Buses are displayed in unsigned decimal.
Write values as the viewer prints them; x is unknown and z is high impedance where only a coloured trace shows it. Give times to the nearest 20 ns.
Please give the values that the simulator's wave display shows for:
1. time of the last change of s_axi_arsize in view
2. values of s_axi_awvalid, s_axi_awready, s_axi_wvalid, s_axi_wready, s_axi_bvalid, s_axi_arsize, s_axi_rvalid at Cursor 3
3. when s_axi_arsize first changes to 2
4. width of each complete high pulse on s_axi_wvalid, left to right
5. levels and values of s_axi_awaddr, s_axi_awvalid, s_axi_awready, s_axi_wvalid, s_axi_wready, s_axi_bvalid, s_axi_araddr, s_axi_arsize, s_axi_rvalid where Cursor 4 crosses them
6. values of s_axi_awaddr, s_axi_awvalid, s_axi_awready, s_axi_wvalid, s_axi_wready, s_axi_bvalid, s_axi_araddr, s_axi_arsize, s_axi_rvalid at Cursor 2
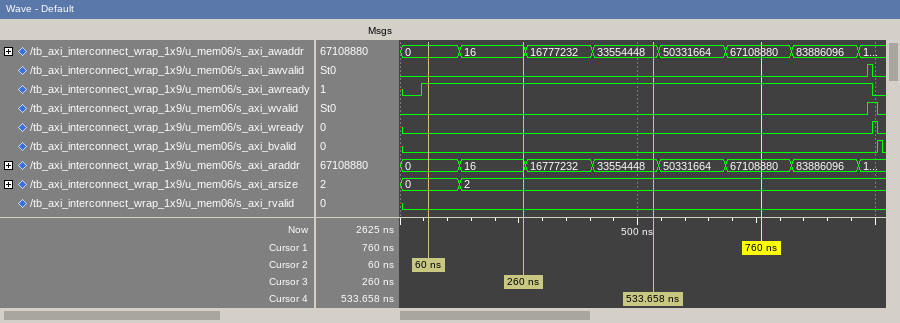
120 ns
s_axi_awvalid=0, s_axi_awready=1, s_axi_wvalid=0, s_axi_wready=0, s_axi_bvalid=0, s_axi_arsize=2, s_axi_rvalid=0
120 ns
20 ns
s_axi_awaddr=33554448, s_axi_awvalid=0, s_axi_awready=1, s_axi_wvalid=0, s_axi_wready=0, s_axi_bvalid=0, s_axi_araddr=33554448, s_axi_arsize=2, s_axi_rvalid=0
s_axi_awaddr=0, s_axi_awvalid=0, s_axi_awready=1, s_axi_wvalid=0, s_axi_wready=0, s_axi_bvalid=0, s_axi_araddr=0, s_axi_arsize=0, s_axi_rvalid=0
